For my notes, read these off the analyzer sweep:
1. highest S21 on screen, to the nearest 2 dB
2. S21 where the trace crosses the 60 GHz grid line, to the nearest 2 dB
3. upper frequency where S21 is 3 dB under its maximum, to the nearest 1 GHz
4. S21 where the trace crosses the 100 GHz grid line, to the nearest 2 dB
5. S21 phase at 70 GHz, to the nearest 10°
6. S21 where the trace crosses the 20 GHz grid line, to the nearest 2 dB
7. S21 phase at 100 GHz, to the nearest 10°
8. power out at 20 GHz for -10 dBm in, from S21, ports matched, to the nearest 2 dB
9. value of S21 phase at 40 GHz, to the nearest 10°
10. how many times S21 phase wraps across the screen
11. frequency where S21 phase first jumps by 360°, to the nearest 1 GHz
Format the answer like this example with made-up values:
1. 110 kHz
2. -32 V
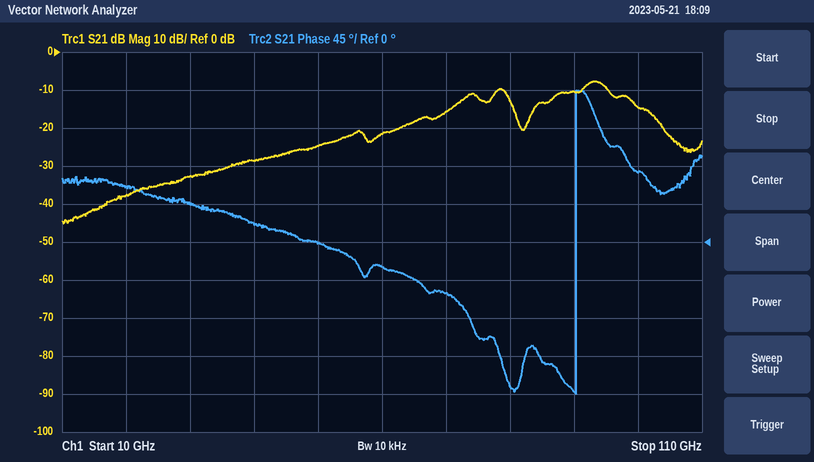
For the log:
1. -8 dB
2. -22 dB
3. 96 GHz
4. -14 dB
5. -60°
6. -38 dB
7. 80°
8. -48 dBm
9. 20°
10. 1
11. 90 GHz
